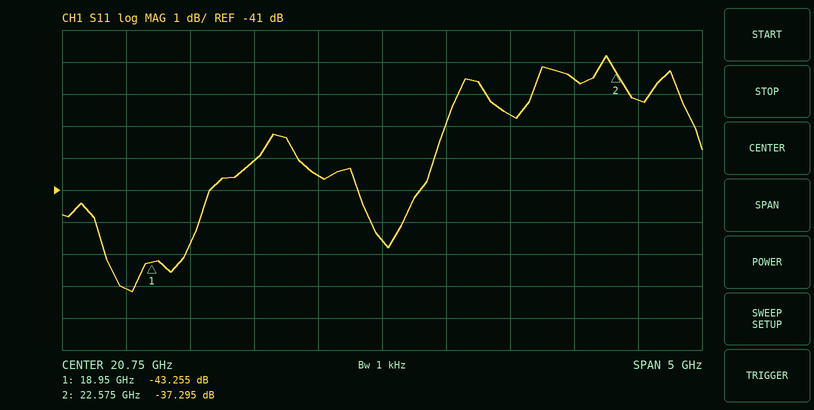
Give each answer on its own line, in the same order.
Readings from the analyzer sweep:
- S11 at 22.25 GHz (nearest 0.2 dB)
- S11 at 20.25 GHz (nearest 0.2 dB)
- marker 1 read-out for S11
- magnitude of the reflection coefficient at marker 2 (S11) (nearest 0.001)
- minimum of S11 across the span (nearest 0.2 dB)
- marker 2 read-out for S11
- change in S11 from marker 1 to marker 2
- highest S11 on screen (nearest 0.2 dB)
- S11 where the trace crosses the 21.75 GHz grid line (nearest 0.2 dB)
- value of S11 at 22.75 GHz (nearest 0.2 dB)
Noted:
-37.6 dB
-40.6 dB
-43.255 dB
0.014
-44.2 dB
-37.295 dB
5.960 dB
-36.8 dB
-38.6 dB
-38.2 dB
